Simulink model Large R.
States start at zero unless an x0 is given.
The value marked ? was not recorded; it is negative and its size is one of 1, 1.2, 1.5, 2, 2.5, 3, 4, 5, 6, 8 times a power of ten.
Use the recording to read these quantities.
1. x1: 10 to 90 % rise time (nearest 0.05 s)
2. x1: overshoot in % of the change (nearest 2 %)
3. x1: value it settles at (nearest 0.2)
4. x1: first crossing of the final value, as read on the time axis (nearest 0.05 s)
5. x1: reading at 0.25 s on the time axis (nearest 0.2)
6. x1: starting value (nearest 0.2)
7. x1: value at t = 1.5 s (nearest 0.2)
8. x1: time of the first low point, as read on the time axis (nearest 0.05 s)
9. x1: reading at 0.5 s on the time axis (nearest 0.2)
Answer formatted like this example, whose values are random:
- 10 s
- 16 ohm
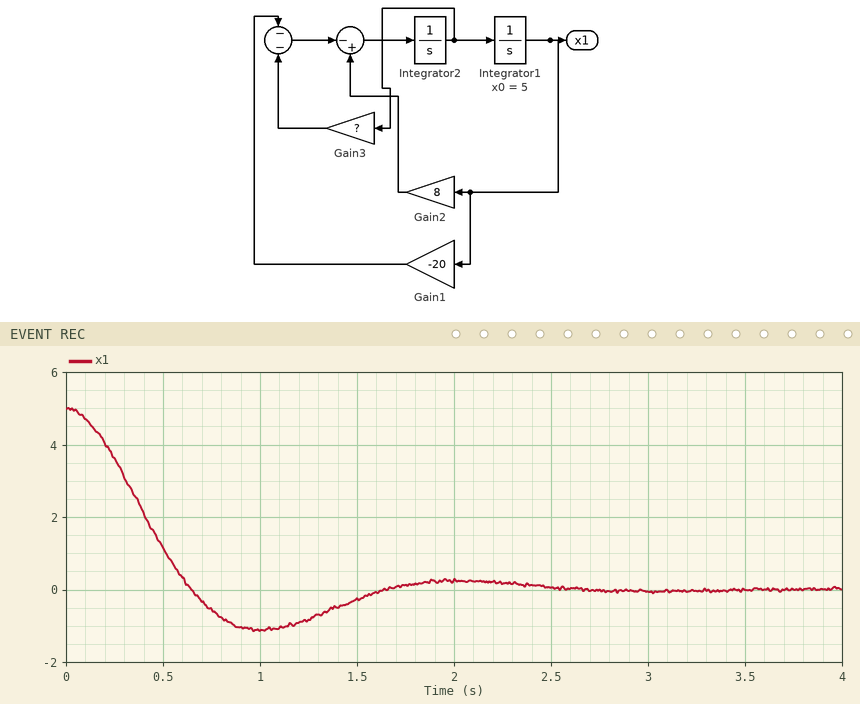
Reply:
- 0.45 s
- 22 %
- 0.0
- 0.65 s
- 3.6
- 5.0
- -0.2
- 1.00 s
- 1.2
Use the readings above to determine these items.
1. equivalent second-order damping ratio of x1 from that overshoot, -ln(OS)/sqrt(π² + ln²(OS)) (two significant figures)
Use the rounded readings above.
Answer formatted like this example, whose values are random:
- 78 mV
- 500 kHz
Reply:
- 0.43
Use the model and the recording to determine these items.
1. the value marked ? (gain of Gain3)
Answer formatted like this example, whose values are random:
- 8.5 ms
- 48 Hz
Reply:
- -3
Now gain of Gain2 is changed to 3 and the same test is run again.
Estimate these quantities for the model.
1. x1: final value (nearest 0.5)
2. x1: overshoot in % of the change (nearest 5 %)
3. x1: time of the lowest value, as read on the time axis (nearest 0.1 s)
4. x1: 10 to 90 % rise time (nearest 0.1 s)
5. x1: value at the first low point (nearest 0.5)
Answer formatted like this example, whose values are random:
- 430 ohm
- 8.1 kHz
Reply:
- 0.0
- 30 %
- 0.8 s
- 0.3 s
- -1.5
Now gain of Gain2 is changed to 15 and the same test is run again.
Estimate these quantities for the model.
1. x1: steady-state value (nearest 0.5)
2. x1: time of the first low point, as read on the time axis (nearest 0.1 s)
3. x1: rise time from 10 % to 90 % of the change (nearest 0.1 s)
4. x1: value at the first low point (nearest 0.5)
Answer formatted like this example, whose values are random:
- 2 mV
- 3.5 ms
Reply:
- 0.0
- 1.9 s
- 0.9 s
- -0.5
